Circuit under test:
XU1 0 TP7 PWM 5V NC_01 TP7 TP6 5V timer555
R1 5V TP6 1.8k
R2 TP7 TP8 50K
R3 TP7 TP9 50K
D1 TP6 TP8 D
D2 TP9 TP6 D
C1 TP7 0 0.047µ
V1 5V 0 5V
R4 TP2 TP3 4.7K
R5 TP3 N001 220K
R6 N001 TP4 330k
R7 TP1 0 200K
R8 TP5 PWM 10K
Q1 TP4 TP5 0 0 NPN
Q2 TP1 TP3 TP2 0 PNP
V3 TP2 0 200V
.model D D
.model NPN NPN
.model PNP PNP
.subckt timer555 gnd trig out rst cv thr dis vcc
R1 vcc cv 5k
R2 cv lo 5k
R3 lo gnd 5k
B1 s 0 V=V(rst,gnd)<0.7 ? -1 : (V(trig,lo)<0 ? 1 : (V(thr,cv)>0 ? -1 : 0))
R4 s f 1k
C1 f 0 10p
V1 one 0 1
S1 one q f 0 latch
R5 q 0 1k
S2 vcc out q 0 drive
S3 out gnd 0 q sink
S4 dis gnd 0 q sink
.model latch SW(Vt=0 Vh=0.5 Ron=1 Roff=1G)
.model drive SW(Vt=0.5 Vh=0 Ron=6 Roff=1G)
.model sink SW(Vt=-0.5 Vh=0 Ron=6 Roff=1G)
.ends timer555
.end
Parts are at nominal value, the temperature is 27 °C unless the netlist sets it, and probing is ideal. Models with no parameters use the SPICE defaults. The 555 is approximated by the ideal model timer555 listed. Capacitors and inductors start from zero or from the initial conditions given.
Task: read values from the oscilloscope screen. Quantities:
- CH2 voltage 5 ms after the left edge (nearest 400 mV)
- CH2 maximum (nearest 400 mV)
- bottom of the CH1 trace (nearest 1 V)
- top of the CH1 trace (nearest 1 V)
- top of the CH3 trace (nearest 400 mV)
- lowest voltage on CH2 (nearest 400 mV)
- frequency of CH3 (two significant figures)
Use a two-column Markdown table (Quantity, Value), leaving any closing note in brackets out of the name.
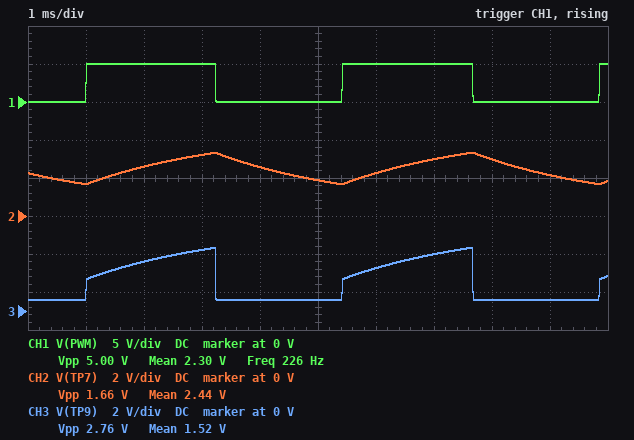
| Quantity | Value |
|---|---|
| CH2 voltage 5 ms after the left edge | 2.0 V |
| CH2 maximum | 3.2 V |
| bottom of the CH1 trace | 0 V |
| top of the CH1 trace | 5 V |
| top of the CH3 trace | 3.2 V |
| lowest voltage on CH2 | 1.6 V |
| frequency of CH3 | 230 Hz |
